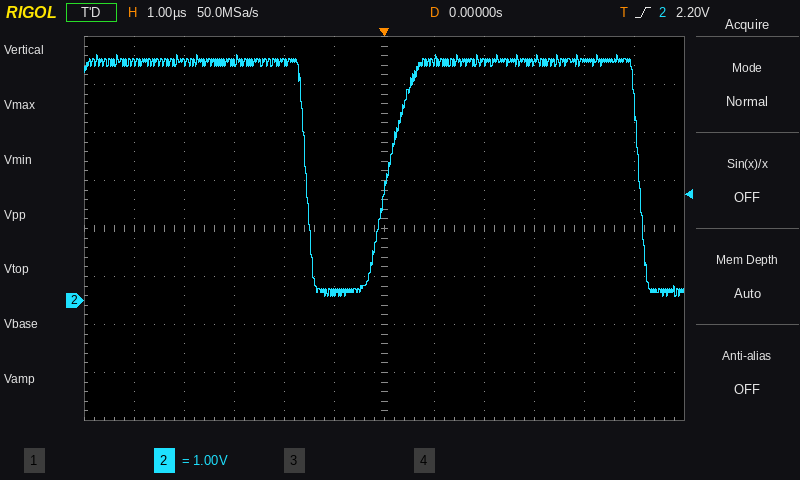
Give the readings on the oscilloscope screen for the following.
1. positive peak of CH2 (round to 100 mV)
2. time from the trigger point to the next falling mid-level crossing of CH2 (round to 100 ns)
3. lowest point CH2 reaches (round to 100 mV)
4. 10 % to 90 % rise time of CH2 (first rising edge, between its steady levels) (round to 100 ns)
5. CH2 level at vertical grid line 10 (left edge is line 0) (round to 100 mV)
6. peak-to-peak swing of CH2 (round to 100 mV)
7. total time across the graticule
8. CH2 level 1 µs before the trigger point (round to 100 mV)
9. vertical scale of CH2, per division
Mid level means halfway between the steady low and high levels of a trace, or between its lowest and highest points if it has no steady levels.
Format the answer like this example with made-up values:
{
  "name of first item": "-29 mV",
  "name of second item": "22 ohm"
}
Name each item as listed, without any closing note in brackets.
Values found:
{
  "positive peak of CH2": "5.1 V",
  "time from the trigger point to the next falling mid-level crossing of CH2": "5.1 µs",
  "lowest point CH2 reaches": "100 mV",
  "10 % to 90 % rise time of CH2 (first rising edge, between its steady levels)": "800 ns",
  "CH2 level at vertical grid line 10 (left edge is line 0)": "5.0 V",
  "peak-to-peak swing of CH2": "5.0 V",
  "total time across the graticule": "12 µs",
  "CH2 level 1 µs before the trigger point": "200 mV",
  "vertical scale of CH2, per division": "1 V"
}
